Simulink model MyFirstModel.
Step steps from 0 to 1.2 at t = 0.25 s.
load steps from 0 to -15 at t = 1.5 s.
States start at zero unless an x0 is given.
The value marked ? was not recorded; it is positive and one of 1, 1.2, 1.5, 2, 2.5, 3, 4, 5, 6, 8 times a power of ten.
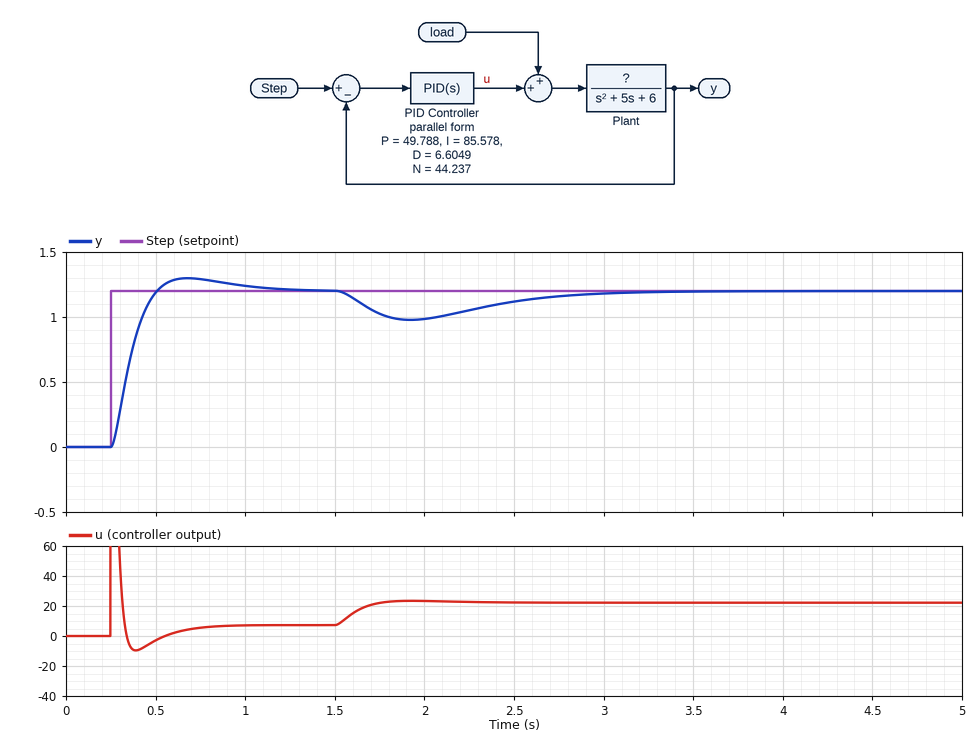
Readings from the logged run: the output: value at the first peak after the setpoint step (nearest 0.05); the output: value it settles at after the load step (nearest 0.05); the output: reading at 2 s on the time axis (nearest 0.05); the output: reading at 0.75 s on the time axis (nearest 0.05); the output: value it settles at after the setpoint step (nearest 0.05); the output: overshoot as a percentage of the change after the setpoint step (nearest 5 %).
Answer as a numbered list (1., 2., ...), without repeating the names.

1. 1.30
2. 1.20
3. 1.00
4. 1.30
5. 1.20
6. 10 %
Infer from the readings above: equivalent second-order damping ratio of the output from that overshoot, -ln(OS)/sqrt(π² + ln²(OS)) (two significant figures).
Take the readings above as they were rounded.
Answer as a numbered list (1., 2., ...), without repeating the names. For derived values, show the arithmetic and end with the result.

1. ln(0.1) = -2.303; 2.303 / sqrt(9.870 + 5.302) = 0.59
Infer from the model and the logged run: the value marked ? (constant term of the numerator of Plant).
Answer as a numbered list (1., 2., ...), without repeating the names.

1. 1
